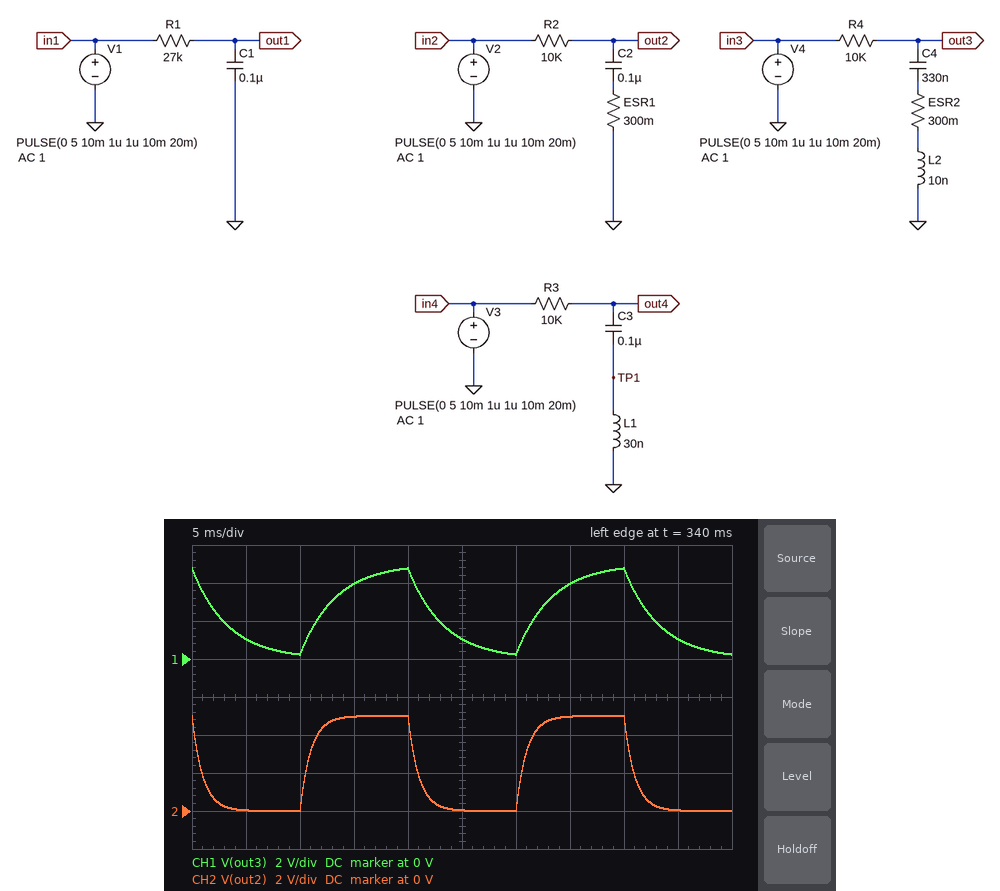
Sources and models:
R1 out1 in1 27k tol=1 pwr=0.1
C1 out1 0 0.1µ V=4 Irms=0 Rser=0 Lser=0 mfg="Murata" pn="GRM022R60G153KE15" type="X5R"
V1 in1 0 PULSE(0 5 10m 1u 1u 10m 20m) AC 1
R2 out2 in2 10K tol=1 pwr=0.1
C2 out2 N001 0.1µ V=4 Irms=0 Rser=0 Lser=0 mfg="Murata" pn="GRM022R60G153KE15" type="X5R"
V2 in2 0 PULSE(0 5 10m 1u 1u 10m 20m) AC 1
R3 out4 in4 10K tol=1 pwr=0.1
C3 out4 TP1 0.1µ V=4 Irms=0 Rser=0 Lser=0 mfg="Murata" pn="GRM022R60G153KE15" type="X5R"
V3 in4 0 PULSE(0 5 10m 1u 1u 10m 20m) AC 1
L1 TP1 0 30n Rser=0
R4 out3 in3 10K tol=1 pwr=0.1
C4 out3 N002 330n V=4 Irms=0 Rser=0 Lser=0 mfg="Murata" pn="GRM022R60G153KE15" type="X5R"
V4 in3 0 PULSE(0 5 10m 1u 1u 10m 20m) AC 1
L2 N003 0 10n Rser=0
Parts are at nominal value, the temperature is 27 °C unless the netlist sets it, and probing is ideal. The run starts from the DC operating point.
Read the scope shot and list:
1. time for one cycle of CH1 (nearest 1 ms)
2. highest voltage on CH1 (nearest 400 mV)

20 ms
4.8 V
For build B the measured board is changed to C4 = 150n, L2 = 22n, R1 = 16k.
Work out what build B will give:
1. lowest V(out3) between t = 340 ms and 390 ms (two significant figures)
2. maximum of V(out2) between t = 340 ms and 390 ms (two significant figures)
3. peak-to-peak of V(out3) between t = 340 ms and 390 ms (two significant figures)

6.4 mV
5.0 V
5.0 V
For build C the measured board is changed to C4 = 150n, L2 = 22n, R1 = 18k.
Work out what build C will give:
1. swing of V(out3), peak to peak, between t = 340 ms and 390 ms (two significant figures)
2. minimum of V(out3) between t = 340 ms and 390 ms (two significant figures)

5.0 V
6.4 mV
